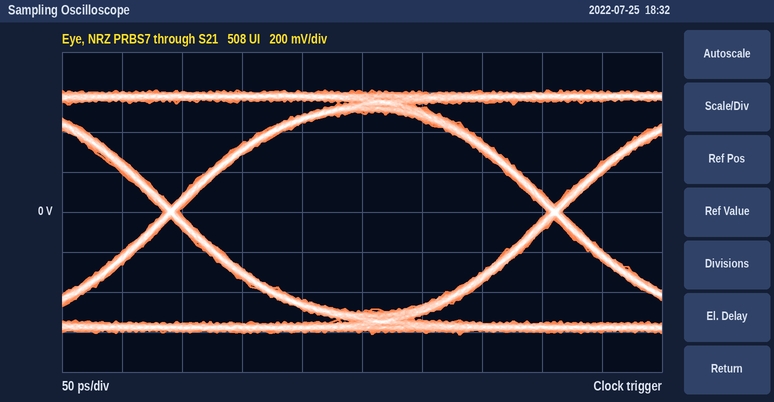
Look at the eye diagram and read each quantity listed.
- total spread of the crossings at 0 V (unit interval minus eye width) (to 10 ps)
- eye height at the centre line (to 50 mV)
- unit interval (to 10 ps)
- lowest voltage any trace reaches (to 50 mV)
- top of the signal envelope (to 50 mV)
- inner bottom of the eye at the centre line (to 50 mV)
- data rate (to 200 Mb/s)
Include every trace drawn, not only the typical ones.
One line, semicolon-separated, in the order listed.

10 ps; 1.00 V; 320 ps; -600 mV; 600 mV; -500 mV; 3.2 Gb/s
